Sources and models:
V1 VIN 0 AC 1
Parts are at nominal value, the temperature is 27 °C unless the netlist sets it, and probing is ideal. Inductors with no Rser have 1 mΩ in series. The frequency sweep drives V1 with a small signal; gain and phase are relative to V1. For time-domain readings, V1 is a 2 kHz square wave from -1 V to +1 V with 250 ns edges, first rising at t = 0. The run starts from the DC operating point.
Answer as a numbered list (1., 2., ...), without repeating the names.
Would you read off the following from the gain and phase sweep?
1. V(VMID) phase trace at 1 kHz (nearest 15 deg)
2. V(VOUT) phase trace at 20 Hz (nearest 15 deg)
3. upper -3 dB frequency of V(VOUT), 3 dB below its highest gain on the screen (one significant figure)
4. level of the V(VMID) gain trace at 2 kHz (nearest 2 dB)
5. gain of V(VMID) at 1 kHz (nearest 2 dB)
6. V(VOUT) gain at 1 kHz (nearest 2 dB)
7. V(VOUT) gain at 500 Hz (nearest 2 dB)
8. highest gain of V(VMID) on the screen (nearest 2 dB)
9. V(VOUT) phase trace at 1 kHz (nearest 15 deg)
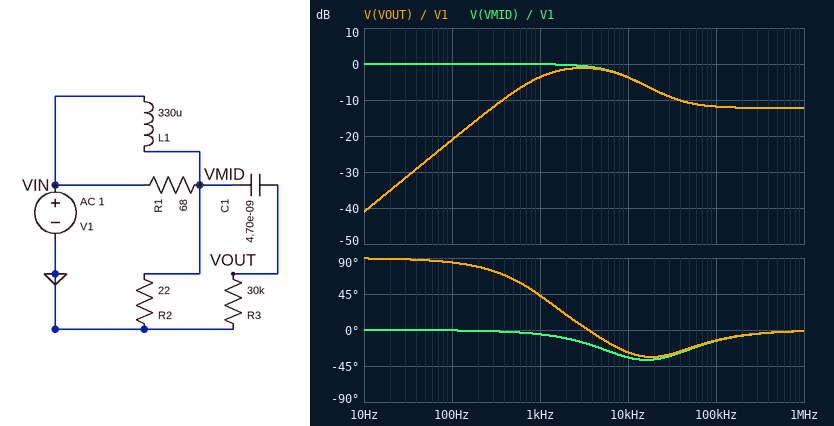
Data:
1. 0 deg
2. 90 deg
3. 10 kHz
4. 0 dB
5. 0 dB
6. -4 dB
7. -8 dB
8. 0 dB
9. 45 deg
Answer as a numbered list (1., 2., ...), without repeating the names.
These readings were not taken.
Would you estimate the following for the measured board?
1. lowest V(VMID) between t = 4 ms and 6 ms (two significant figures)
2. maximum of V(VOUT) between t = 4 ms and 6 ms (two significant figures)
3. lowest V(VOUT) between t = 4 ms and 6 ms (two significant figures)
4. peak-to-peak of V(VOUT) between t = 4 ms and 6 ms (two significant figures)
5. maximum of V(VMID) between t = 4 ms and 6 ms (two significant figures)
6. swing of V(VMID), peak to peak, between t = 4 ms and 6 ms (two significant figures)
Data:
1. -1.0 V
2. 1.2 V
3. -1.2 V
4. 2.4 V
5. 1.0 V
6. 2.0 V
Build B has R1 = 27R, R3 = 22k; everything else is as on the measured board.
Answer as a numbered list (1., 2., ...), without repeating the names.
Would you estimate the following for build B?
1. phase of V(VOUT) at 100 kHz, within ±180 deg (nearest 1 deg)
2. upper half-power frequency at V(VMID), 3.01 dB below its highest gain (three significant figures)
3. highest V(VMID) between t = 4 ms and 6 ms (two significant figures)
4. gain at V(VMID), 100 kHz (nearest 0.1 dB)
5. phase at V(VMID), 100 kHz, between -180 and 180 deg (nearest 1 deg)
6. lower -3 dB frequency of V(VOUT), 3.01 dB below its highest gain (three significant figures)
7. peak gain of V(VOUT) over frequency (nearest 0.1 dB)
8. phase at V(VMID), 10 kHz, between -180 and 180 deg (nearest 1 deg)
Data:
1. -3 deg
2. 7.56 kHz
3. 1.0 V
4. -6.9 dB
5. -4 deg
6. 1.11 kHz
7. -1.8 dB
8. -22 deg
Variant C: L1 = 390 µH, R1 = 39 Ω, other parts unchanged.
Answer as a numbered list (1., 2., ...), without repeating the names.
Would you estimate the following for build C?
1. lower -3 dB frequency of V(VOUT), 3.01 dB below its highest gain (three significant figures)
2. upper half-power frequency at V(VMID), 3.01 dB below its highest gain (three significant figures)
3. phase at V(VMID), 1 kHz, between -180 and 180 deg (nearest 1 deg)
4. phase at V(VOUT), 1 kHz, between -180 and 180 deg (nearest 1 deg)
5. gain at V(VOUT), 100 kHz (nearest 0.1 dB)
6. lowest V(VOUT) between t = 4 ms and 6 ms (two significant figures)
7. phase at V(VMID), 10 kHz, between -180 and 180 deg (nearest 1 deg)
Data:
1. 857 Hz
2. 6.67 kHz
3. -6 deg
4. 42 deg
5. -8.8 dB
6. -1.1 V
7. -28 deg
